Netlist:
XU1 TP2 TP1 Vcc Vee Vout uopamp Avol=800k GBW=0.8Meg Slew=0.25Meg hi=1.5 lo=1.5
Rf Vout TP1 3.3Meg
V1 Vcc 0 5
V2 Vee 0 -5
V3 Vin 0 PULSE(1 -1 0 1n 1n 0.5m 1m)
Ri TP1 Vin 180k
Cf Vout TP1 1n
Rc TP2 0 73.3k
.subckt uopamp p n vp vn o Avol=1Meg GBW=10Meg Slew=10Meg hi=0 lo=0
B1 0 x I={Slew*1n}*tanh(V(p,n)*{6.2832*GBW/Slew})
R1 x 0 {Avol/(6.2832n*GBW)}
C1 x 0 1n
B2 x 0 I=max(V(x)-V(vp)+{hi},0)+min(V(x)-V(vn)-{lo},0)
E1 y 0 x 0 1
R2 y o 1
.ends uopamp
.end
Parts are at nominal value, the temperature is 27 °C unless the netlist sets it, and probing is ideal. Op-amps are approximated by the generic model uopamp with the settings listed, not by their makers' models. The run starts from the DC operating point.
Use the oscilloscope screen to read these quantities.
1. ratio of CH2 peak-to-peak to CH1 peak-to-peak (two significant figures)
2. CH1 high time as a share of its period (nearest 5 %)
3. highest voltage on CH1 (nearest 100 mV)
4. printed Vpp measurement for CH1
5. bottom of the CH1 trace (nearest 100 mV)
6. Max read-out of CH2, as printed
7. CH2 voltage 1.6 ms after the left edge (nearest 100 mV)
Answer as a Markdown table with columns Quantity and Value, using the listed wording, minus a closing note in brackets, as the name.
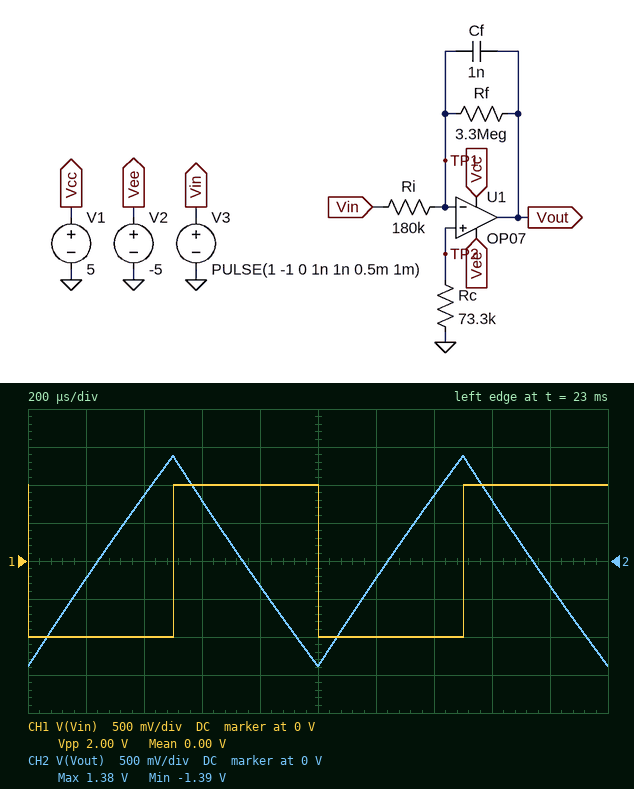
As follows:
| Quantity | Value |
|---|---|
| ratio of CH2 peak-to-peak to CH1 peak-to-peak | 1.4 |
| CH1 high time as a share of its period | 50 % |
| highest voltage on CH1 | 1.0 V |
| printed Vpp measurement for CH1 | 2.00 V |
| bottom of the CH1 trace | -1.0 V |
| Max read-out of CH2, as printed | 1.38 V |
| CH2 voltage 1.6 ms after the left edge | 800 mV |
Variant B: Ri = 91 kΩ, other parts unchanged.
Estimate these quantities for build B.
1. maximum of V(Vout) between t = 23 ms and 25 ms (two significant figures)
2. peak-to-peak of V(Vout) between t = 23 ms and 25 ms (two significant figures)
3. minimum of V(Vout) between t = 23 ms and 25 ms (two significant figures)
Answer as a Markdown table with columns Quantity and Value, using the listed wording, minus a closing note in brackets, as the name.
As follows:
| Quantity | Value |
|---|---|
| maximum of V(Vout) between t = 23 ms and 25 ms | 2.7 V |
| peak-to-peak of V(Vout) between t = 23 ms and 25 ms | 5.5 V |
| minimum of V(Vout) between t = 23 ms and 25 ms | -2.7 V |
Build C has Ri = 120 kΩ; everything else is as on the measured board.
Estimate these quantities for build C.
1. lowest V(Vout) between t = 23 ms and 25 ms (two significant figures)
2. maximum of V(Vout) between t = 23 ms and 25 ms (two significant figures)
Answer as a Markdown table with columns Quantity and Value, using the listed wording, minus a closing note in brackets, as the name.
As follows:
| Quantity | Value |
|---|---|
| lowest V(Vout) between t = 23 ms and 25 ms | -2.1 V |
| maximum of V(Vout) between t = 23 ms and 25 ms | 2.1 V |
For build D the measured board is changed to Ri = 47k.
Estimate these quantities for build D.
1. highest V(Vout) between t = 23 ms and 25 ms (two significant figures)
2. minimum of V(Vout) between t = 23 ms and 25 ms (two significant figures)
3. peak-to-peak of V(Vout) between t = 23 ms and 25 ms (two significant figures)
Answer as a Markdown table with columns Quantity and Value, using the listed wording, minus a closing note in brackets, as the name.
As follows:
| Quantity | Value |
|---|---|
| highest V(Vout) between t = 23 ms and 25 ms | 3.5 V |
| minimum of V(Vout) between t = 23 ms and 25 ms | -3.5 V |
| peak-to-peak of V(Vout) between t = 23 ms and 25 ms | 7.0 V |
